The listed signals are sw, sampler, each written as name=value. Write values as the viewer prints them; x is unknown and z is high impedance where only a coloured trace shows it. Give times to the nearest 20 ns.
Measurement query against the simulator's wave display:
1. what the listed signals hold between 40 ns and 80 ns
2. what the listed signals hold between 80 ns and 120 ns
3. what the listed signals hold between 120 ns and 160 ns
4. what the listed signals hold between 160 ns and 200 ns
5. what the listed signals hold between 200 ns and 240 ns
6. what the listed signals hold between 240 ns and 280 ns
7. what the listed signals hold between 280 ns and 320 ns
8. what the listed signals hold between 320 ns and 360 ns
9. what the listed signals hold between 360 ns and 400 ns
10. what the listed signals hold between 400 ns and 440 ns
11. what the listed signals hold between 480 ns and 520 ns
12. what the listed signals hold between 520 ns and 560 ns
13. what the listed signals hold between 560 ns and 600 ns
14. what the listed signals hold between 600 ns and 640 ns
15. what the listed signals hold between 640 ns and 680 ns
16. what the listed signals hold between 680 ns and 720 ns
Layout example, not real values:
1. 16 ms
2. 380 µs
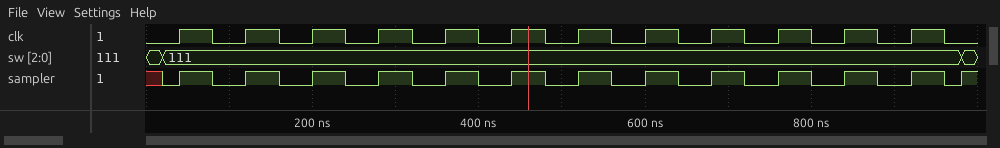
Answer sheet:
1. sw=111, sampler=1
2. sw=111, sampler=0
3. sw=111, sampler=1
4. sw=111, sampler=0
5. sw=111, sampler=1
6. sw=111, sampler=0
7. sw=111, sampler=1
8. sw=111, sampler=0
9. sw=111, sampler=1
10. sw=111, sampler=0
11. sw=111, sampler=0
12. sw=111, sampler=1
13. sw=111, sampler=0
14. sw=111, sampler=1
15. sw=111, sampler=0
16. sw=111, sampler=1
